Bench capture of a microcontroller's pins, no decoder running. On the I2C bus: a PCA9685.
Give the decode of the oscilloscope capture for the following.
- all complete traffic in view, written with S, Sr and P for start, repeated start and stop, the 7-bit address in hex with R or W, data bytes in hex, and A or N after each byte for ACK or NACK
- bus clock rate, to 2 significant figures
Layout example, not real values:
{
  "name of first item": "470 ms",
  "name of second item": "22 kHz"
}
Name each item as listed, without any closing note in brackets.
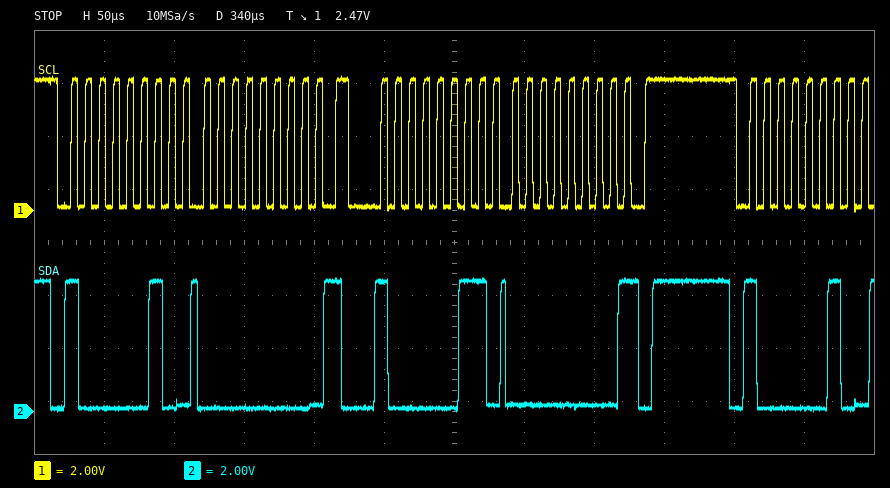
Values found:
{
  "all complete traffic in view, written with S, Sr and P for start, repeated start and stop, the 7-bit address in hex with R or W, data bytes in hex, and A or N after each byte for ACK or NACK": "S 41W A 00 A Sr 41R A 00 N P S 41W A",
  "bus clock rate, to 2 significant figures": "100 kHz"
}
